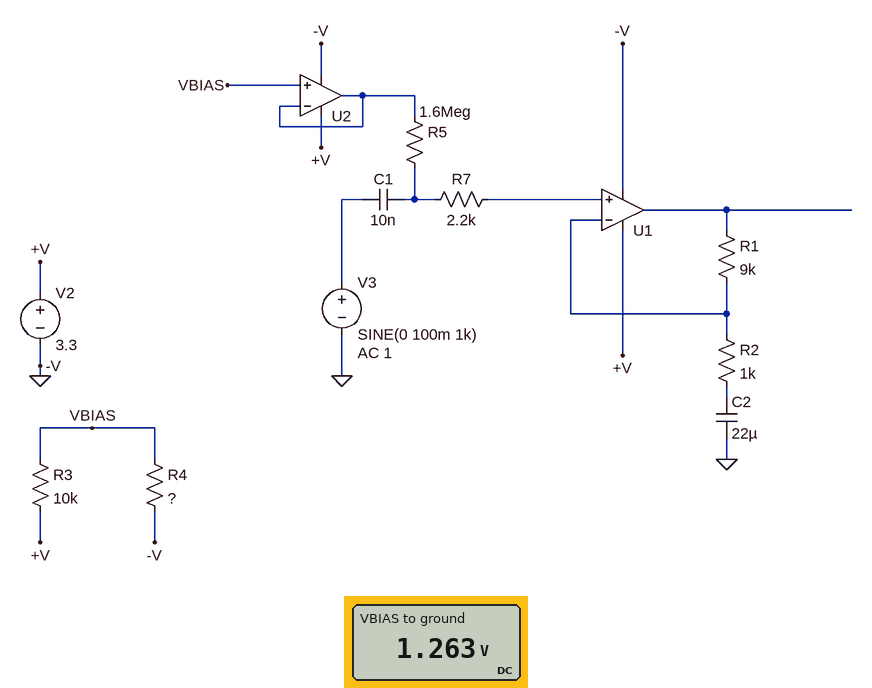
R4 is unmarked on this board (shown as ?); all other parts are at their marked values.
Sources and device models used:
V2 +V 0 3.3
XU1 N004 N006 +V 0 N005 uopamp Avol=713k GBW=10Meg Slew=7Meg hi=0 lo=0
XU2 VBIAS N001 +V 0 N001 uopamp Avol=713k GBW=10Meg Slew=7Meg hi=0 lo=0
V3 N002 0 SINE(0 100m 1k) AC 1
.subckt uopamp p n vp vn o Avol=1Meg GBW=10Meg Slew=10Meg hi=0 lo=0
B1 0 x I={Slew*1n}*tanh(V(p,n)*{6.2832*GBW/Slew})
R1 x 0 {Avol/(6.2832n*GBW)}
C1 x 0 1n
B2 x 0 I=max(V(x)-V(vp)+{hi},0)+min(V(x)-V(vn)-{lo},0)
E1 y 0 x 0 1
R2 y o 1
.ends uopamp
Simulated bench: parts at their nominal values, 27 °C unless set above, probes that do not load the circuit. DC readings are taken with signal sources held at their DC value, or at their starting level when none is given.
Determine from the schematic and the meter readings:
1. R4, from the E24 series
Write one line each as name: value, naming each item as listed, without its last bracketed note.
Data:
R4, from the E24 series: 6.2 kΩ
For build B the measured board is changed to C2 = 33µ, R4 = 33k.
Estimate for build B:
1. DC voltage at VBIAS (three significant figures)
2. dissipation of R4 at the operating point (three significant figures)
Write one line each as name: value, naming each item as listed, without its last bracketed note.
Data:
DC voltage at VBIAS: 2.53 V
dissipation of R4 at the operating point: 194 µW
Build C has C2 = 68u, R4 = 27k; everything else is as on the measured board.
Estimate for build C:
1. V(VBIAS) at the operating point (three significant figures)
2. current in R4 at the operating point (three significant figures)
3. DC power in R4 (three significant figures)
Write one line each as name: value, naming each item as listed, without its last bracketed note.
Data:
V(VBIAS) at the operating point: 2.41 V
current in R4 at the operating point: 89.2 µA
DC power in R4: 215 µW
